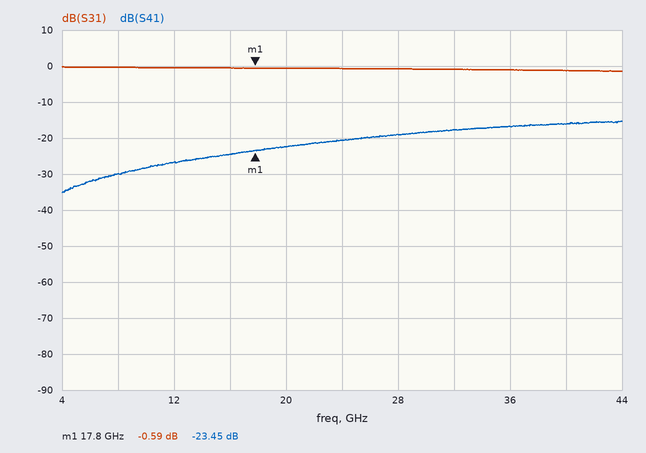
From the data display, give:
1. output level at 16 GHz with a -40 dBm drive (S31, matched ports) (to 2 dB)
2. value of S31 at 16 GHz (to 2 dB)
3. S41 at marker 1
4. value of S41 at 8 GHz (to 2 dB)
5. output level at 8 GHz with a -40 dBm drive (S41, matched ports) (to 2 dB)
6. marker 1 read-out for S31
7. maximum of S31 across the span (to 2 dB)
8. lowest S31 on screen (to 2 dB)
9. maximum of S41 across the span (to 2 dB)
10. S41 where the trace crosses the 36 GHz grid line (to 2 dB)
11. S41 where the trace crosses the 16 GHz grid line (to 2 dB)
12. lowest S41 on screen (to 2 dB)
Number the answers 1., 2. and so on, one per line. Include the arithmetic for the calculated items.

1. -40 dBm + (0 dB) = -40 dBm
2. 0 dB
3. -23.45 dB
4. -30 dB
5. -40 dBm + (-30 dB) = -70 dBm
6. -0.59 dB
7. 0 dB
8. -2 dB
9. -16 dB
10. -16 dB
11. -24 dB
12. -36 dB
